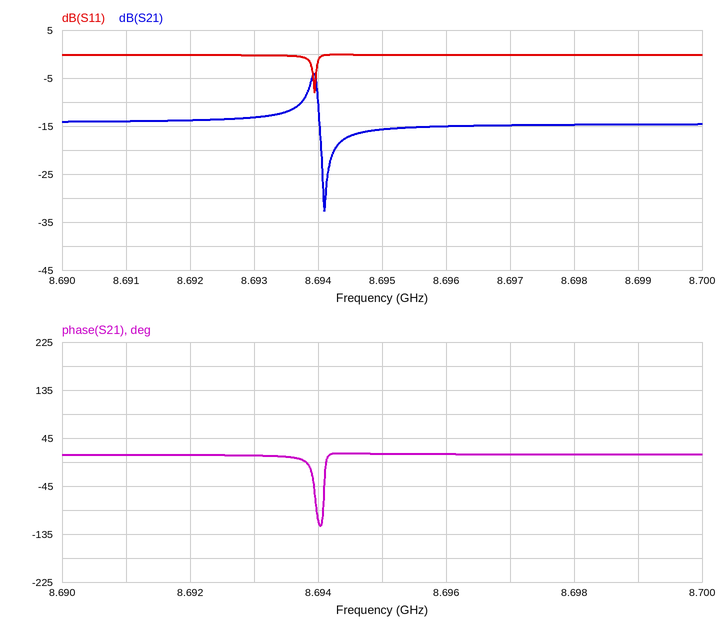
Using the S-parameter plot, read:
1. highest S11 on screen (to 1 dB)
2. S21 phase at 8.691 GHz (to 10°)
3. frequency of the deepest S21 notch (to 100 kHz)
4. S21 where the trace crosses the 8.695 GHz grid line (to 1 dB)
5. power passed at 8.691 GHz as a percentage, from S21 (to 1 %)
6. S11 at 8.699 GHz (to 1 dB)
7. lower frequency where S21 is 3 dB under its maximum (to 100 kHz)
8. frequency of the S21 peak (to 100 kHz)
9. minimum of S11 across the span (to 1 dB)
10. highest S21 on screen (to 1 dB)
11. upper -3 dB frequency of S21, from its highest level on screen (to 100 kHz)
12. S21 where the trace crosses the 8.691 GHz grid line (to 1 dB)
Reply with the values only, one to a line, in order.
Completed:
0 dB
10°
8.6941 GHz
-16 dB
4 %
0 dB
8.6939 GHz
8.6939 GHz
-8 dB
-4 dB
8.6940 GHz
-14 dB
